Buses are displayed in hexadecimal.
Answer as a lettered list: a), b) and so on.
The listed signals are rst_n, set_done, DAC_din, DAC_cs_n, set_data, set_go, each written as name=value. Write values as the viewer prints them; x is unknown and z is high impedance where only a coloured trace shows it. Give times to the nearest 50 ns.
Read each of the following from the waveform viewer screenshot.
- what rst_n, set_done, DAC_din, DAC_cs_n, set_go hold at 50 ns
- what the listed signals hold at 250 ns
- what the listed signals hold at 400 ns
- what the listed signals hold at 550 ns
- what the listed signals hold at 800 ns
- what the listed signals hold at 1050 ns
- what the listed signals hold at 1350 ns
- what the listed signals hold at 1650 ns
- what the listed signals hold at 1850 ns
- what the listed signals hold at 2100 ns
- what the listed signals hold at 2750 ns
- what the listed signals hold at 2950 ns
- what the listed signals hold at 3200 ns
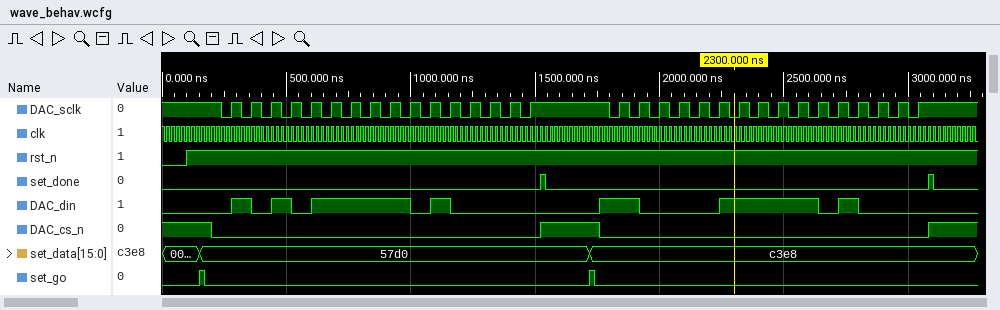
a) rst_n=0, set_done=0, DAC_din=0, DAC_cs_n=1, set_go=0
b) rst_n=1, set_done=0, DAC_din=0, DAC_cs_n=0, set_data=57d0, set_go=0
c) rst_n=1, set_done=0, DAC_din=0, DAC_cs_n=0, set_data=57d0, set_go=0
d) rst_n=1, set_done=0, DAC_din=0, DAC_cs_n=0, set_data=57d0, set_go=0
e) rst_n=1, set_done=0, DAC_din=1, DAC_cs_n=0, set_data=57d0, set_go=0
f) rst_n=1, set_done=0, DAC_din=0, DAC_cs_n=0, set_data=57d0, set_go=0
g) rst_n=1, set_done=0, DAC_din=0, DAC_cs_n=0, set_data=57d0, set_go=0
h) rst_n=1, set_done=0, DAC_din=0, DAC_cs_n=1, set_data=57d0, set_go=0
i) rst_n=1, set_done=0, DAC_din=1, DAC_cs_n=0, set_data=c3e8, set_go=0
j) rst_n=1, set_done=0, DAC_din=0, DAC_cs_n=0, set_data=c3e8, set_go=0
k) rst_n=1, set_done=0, DAC_din=1, DAC_cs_n=0, set_data=c3e8, set_go=0
l) rst_n=1, set_done=0, DAC_din=0, DAC_cs_n=0, set_data=c3e8, set_go=0
m) rst_n=1, set_done=0, DAC_din=0, DAC_cs_n=1, set_data=c3e8, set_go=0
